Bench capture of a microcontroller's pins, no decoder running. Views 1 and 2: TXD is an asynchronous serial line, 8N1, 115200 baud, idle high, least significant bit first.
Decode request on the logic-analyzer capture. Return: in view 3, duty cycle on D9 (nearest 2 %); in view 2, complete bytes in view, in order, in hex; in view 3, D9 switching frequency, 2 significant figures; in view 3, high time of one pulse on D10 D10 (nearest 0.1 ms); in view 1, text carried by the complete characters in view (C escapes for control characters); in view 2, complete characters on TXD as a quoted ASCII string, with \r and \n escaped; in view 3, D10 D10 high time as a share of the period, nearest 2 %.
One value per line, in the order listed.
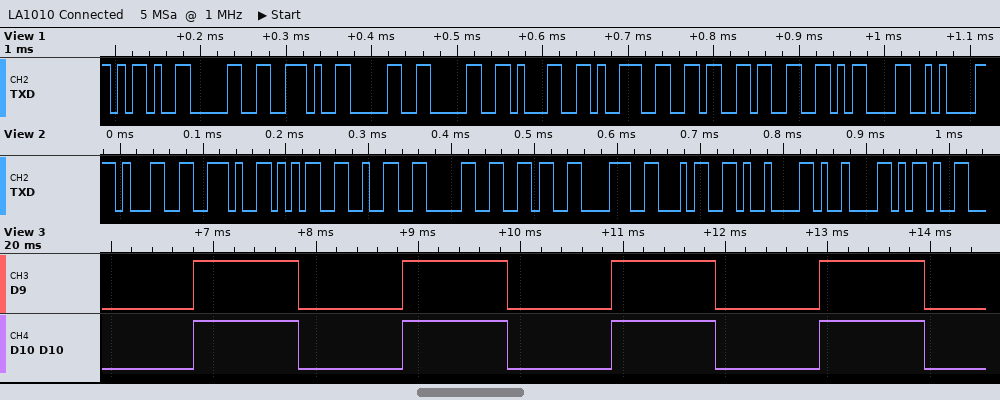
50 %
31 2E 35 32 30 36 38 34 09 09 2D
490 Hz
1.0 ms
"-0.001963\r\n"
"1.520684\t\t-"
50 %
